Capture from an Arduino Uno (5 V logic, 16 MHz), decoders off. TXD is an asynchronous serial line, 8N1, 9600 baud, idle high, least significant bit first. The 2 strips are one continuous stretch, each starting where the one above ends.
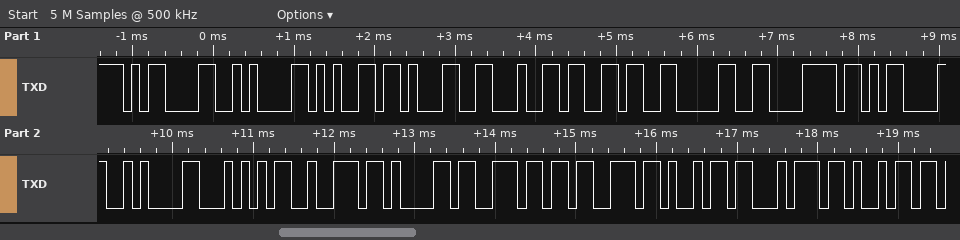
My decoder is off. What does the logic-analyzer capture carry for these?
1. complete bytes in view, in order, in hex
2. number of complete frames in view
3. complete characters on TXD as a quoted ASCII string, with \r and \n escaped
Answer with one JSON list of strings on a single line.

["0x0D 0x0A 0x65 0x31 0x64 0x36 0x30 0x78 0x0D 0x0A 0x54 0x72 0x61 0x6E 0x73 0x69 0x74 0x69", "18", "\"\\r\\ne1d60x\\r\\nTransiti\""]
